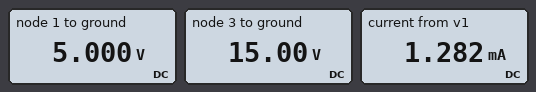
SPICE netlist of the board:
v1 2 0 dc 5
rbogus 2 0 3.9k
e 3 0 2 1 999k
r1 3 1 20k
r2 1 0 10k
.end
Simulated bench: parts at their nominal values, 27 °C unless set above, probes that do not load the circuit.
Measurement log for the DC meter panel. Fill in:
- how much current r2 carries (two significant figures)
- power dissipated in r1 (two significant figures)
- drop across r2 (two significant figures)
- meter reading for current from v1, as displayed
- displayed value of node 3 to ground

500 µA
5.0 mW
5.0 V
1.282 mA
15.00 V
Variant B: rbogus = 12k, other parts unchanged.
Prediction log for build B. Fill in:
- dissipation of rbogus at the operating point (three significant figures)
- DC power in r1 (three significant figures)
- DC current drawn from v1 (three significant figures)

2.08 mW
5.00 mW
417 µA
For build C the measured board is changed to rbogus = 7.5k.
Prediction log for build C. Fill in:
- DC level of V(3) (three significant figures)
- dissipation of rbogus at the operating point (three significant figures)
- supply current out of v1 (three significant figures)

15.0 V
3.33 mW
667 µA
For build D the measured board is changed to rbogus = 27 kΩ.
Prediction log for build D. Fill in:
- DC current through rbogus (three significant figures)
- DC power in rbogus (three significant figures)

185 µA
926 µW
